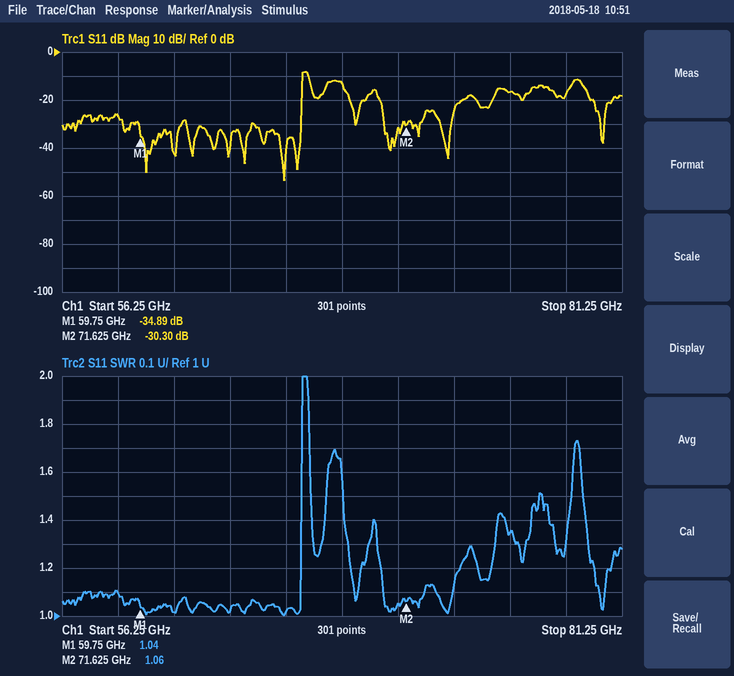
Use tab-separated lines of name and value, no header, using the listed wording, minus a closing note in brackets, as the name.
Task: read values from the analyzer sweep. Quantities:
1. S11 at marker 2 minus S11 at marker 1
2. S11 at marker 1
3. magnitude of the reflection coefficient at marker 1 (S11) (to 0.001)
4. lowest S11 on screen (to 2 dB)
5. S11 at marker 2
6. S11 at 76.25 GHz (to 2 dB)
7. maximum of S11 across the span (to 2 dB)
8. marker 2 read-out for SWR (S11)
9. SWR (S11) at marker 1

S11 at marker 2 minus S11 at marker 1	4.59 dB
S11 at marker 1	-34.89 dB
magnitude of the reflection coefficient at marker 1 (S11)	0.018
lowest S11 on screen	-54 dB
S11 at marker 2	-30.30 dB
S11 at 76.25 GHz	-16 dB
maximum of S11 across the span	-8 dB
marker 2 read-out for SWR	1.06
SWR (S11) at marker 1	1.04
